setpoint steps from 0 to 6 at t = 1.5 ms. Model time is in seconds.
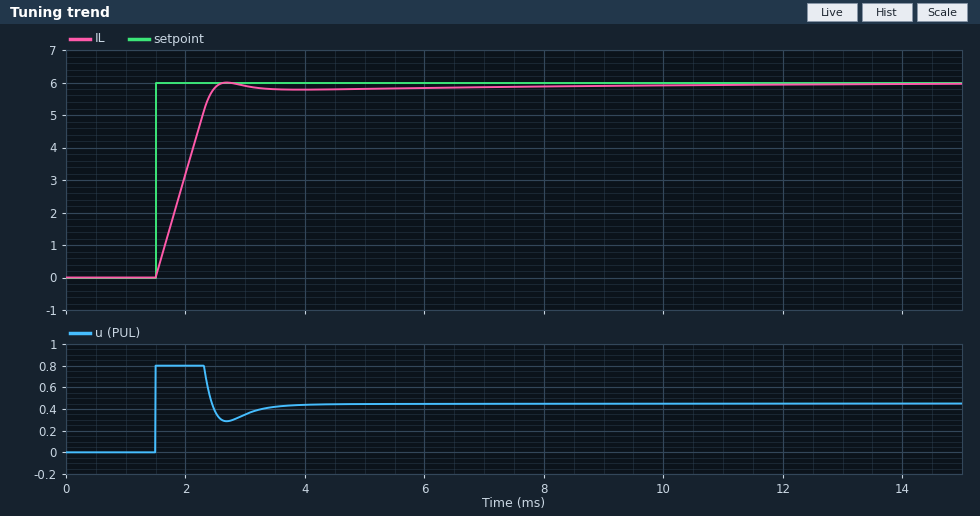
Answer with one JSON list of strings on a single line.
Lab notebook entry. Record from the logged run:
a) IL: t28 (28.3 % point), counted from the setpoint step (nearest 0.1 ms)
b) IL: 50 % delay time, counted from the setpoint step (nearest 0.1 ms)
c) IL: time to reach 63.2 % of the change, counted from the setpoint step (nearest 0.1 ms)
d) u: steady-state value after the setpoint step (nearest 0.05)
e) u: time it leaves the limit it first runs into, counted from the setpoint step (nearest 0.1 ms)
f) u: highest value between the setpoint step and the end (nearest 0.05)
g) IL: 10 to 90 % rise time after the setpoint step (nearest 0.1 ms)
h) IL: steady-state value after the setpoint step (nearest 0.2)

["0.3 ms", "0.5 ms", "0.6 ms", "0.45", "0.8 ms", "0.80", "0.8 ms", "6.0"]
